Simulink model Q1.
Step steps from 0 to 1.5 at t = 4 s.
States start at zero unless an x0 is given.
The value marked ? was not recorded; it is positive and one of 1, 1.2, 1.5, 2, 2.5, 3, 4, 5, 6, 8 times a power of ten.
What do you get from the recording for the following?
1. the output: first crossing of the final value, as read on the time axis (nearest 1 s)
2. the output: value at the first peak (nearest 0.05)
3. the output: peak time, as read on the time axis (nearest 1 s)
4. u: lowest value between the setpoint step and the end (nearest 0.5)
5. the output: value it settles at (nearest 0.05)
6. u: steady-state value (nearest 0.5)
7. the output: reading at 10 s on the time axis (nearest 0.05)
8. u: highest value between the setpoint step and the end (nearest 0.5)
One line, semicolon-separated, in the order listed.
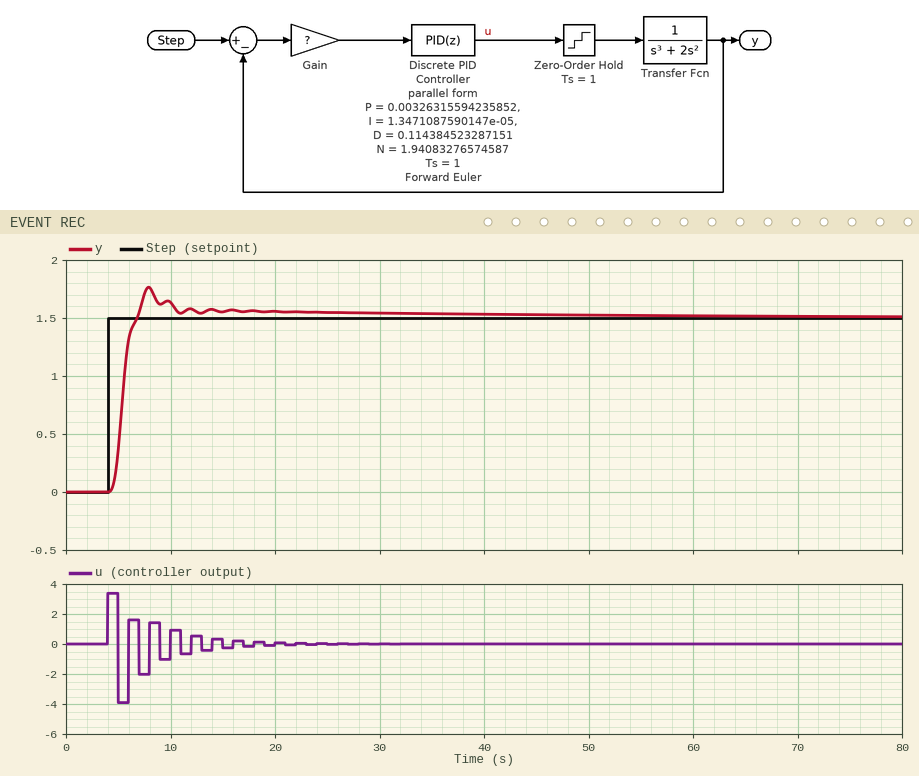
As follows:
7 s; 1.75; 8 s; -4.0; 1.50; 0.0; 1.65; 3.5
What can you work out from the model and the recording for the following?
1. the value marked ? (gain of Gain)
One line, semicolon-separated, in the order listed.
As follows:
10
